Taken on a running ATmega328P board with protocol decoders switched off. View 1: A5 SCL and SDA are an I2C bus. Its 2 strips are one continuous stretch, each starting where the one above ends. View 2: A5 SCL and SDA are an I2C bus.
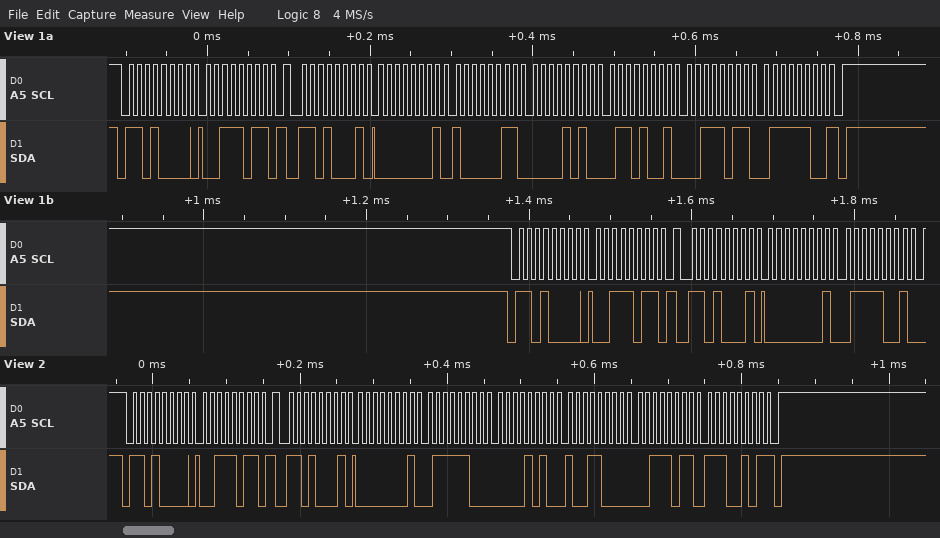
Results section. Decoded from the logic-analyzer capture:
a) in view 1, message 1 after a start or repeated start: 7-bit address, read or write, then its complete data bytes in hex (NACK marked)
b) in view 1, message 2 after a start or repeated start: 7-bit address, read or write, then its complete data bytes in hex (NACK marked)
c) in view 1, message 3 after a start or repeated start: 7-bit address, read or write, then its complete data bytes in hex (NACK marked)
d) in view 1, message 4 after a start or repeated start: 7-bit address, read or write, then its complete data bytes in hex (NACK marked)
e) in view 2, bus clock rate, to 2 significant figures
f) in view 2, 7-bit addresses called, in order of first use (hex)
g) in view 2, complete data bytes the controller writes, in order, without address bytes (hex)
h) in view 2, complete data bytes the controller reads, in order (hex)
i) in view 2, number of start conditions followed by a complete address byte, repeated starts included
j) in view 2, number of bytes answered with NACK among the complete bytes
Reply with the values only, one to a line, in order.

0x68 write: 3B
0x68 read: 01 83 0A 69 3B 7C NACK
0x68 write: 3B
0x68 read: 01 79
100 kHz
0x68
3B
01 7C 0A 98 3B E5
2
1
